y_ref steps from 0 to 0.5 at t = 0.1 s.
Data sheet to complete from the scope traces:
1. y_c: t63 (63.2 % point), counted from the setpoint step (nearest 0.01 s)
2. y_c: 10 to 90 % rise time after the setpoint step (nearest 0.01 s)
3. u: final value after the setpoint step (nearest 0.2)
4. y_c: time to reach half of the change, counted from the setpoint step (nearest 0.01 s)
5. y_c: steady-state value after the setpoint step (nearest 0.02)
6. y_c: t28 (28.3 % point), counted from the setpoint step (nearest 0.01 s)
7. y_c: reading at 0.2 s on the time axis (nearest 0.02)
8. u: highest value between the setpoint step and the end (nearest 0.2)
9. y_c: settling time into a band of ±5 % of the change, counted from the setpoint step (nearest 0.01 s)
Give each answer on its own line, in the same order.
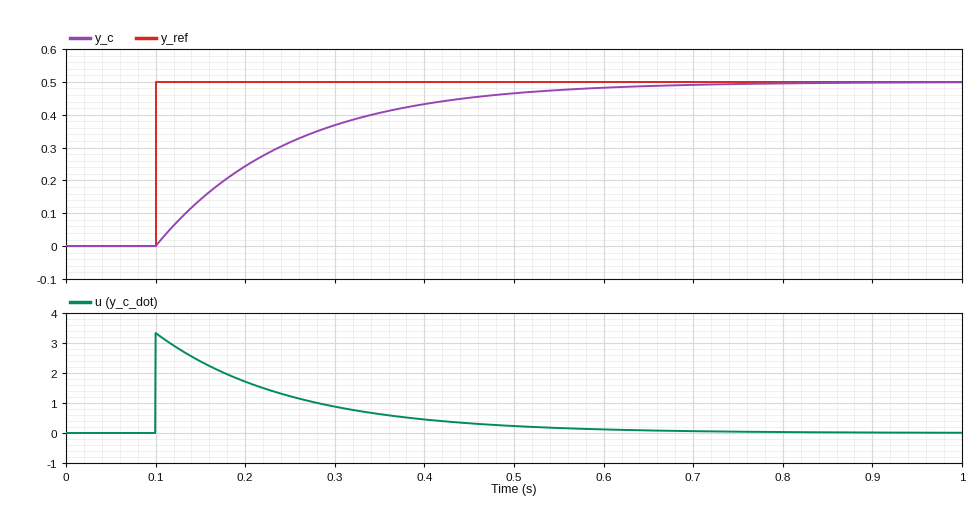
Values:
0.15 s
0.33 s
0.0
0.10 s
0.50
0.05 s
0.24
3.4
0.45 s
